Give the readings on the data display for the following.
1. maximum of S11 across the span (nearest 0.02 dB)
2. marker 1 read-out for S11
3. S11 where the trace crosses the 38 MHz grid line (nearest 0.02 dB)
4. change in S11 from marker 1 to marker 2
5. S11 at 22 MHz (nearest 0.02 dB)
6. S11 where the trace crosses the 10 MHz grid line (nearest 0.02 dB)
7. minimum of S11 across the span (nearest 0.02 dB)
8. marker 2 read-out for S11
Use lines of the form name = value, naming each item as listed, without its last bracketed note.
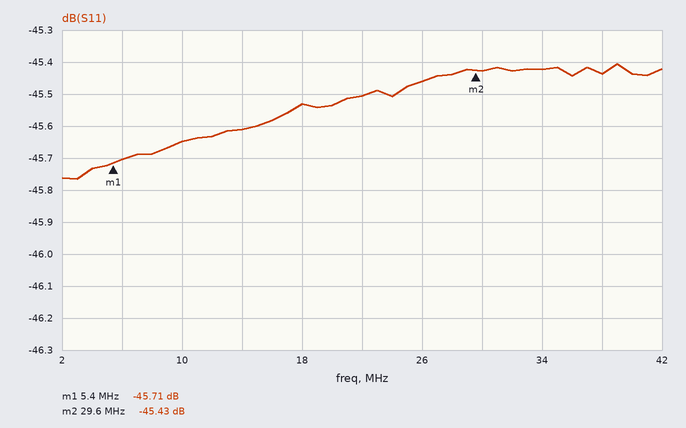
maximum of S11 across the span = -45.40 dB
marker 1 read-out for S11 = -45.71 dB
S11 where the trace crosses the 38 MHz grid line = -45.44 dB
change in S11 from marker 1 to marker 2 = 0.28 dB
S11 at 22 MHz = -45.50 dB
S11 where the trace crosses the 10 MHz grid line = -45.64 dB
minimum of S11 across the span = -45.76 dB
marker 2 read-out for S11 = -45.43 dB
